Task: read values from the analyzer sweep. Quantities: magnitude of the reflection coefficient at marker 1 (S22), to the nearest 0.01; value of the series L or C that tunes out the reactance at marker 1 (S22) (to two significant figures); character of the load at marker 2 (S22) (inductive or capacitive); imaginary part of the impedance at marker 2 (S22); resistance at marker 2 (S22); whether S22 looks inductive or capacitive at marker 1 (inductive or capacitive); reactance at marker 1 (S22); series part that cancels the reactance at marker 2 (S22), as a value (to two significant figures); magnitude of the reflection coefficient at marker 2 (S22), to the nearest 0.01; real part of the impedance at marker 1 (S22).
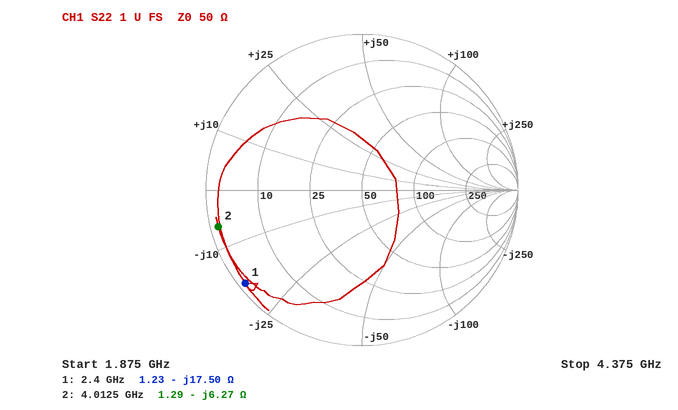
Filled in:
0.96
1.2 nH
capacitive
-6.27 Ω
1.29 Ω
capacitive
-17.50 Ω
250 pH
0.95
1.23 Ω
